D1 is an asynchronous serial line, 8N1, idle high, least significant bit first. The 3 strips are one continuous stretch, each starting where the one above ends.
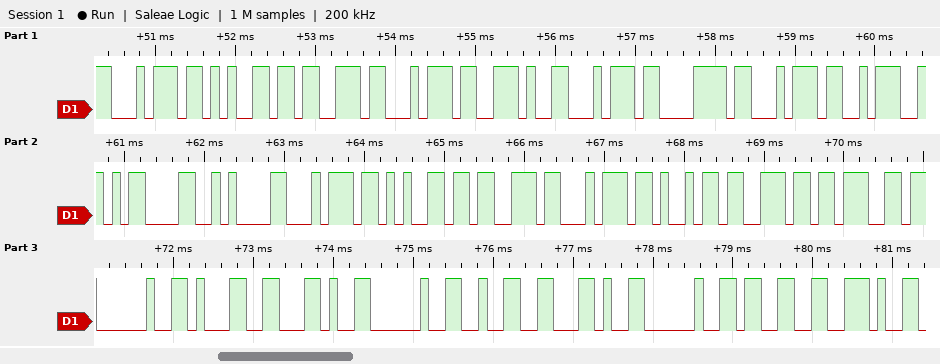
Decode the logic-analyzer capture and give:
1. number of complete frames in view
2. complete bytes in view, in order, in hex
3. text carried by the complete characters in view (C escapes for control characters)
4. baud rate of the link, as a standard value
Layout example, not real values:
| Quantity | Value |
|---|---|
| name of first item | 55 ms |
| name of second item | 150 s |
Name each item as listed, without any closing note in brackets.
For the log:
| Quantity | Value |
|---|---|
| number of complete frames in view | 27 |
| complete bytes in view, in order, in hex | 74 65 73 74 2E 74 78 74 3A 0D 0A 74 65 73 74 69 6E 67 20 31 2C 20 32 2C 20 33 2E |
| text carried by the complete characters in view | "test.txt:\r\ntesting 1, 2, 3." |
| baud rate of the link, as a standard value | 9600 baud |
